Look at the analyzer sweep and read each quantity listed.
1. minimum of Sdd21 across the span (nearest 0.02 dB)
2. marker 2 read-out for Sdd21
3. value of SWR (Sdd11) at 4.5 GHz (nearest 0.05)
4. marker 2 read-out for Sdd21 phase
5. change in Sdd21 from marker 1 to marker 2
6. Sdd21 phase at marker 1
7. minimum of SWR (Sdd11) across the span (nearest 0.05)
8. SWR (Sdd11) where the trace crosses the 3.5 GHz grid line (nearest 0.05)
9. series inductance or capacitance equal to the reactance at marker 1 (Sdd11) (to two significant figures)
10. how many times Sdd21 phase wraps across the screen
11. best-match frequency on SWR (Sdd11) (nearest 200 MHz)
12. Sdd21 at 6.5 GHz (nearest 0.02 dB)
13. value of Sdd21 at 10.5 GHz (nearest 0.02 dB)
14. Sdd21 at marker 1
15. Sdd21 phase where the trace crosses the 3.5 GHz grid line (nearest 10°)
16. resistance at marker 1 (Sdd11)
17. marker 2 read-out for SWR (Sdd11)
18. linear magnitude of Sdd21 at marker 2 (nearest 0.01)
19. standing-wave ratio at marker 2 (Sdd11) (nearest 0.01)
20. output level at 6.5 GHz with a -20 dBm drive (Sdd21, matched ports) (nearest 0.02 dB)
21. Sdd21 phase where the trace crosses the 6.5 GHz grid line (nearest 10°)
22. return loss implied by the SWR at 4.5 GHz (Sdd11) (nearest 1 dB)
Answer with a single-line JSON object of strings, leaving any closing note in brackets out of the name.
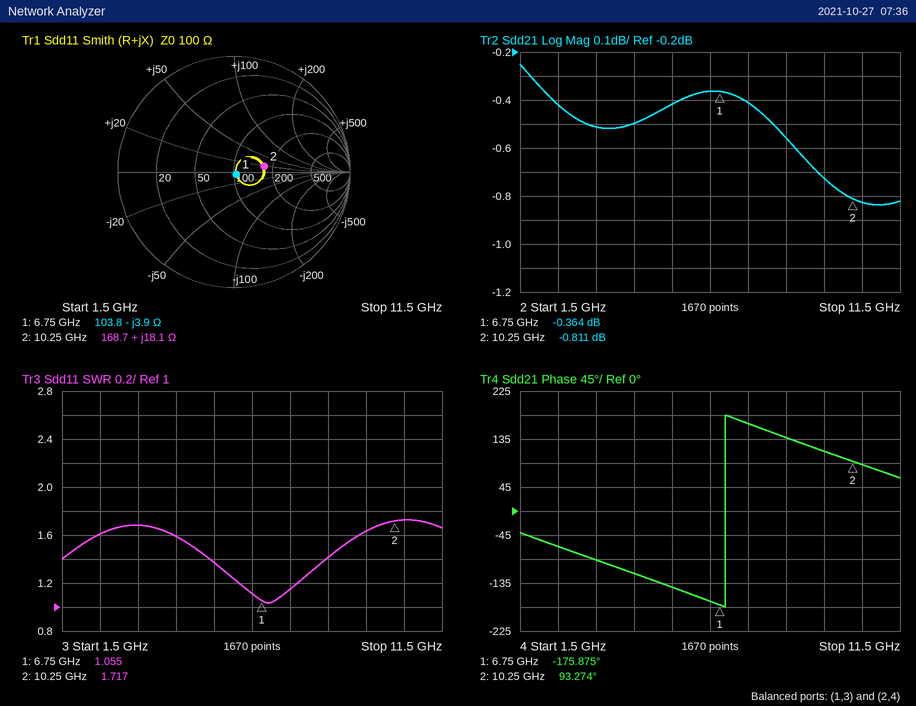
{"minimum of Sdd21 across the span": "-0.84 dB", "marker 2 read-out for Sdd21": "-0.811 dB", "value of SWR (Sdd11) at 4.5 GHz": "1.60", "marker 2 read-out for Sdd21 phase": "93.274°", "change in Sdd21 from marker 1 to marker 2": "-0.447 dB", "Sdd21 phase at marker 1": "-175.875°", "minimum of SWR (Sdd11) across the span": "1.05", "SWR (Sdd11) where the trace crosses the 3.5 GHz grid line": "1.70", "series inductance or capacitance equal to the reactance at marker 1 (Sdd11)": "6.0 pF", "how many times Sdd21 phase wraps across the screen": "1", "best-match frequency on SWR (Sdd11)": "7.0 GHz", "Sdd21 at 6.5 GHz": "-0.36 dB", "value of Sdd21 at 10.5 GHz": "-0.82 dB", "Sdd21 at marker 1": "-0.364 dB", "Sdd21 phase where the trace crosses the 3.5 GHz grid line": "-90°", "resistance at marker 1": "103.8 Ω", "marker 2 read-out for SWR": "1.717", "linear magnitude of Sdd21 at marker 2": "0.91", "standing-wave ratio at marker 2 (Sdd11)": "1.72", "output level at 6.5 GHz with a -20 dBm drive (Sdd21, matched ports)": "-20.36 dBm", "Sdd21 phase where the trace crosses the 6.5 GHz grid line": "-170°", "return loss implied by the SWR at 4.5 GHz (Sdd11)": "13 dB"}
